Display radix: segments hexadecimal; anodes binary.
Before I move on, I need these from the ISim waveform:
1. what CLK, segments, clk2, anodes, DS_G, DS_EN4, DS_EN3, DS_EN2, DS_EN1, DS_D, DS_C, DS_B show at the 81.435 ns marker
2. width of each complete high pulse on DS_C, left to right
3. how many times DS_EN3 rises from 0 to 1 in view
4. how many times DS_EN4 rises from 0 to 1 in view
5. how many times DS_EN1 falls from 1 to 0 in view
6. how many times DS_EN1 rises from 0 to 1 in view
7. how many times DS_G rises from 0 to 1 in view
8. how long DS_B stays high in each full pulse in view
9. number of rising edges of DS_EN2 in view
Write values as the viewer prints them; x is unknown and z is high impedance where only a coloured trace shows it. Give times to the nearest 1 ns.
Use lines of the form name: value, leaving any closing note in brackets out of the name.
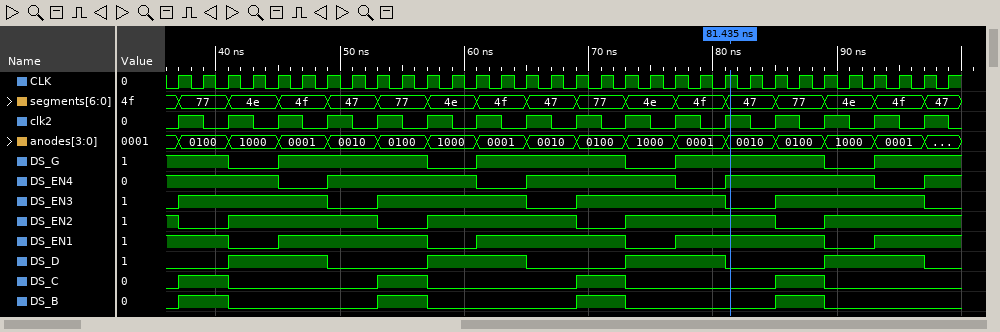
what CLK, segments, clk2, anodes, DS_G, DS_EN4, DS_EN3, DS_EN2, DS_EN1, DS_D, DS_C, DS_B show at the 81.435 ns marker: CLK=1, segments=47, clk2=1, anodes=0010, DS_G=1, DS_EN4=1, DS_EN3=0, DS_EN2=1, DS_EN1=1, DS_D=0, DS_C=0, DS_B=0
width of each complete high pulse on DS_C, left to right: 4 ns, 4 ns, 4 ns, 4 ns
how many times DS_EN3 rises from 0 to 1 in view: 4
how many times DS_EN4 rises from 0 to 1 in view: 4
how many times DS_EN1 falls from 1 to 0 in view: 4
how many times DS_EN1 rises from 0 to 1 in view: 4
how many times DS_G rises from 0 to 1 in view: 4
how long DS_B stays high in each full pulse in view: 4 ns, 4 ns, 4 ns, 4 ns
number of rising edges of DS_EN2 in view: 4
